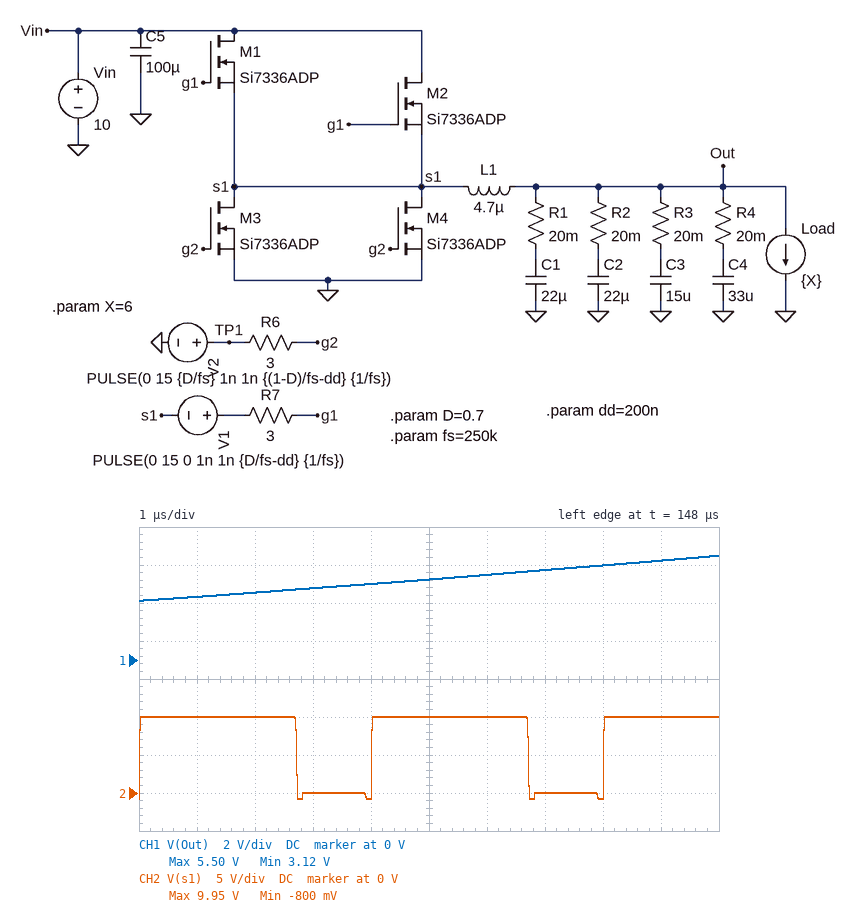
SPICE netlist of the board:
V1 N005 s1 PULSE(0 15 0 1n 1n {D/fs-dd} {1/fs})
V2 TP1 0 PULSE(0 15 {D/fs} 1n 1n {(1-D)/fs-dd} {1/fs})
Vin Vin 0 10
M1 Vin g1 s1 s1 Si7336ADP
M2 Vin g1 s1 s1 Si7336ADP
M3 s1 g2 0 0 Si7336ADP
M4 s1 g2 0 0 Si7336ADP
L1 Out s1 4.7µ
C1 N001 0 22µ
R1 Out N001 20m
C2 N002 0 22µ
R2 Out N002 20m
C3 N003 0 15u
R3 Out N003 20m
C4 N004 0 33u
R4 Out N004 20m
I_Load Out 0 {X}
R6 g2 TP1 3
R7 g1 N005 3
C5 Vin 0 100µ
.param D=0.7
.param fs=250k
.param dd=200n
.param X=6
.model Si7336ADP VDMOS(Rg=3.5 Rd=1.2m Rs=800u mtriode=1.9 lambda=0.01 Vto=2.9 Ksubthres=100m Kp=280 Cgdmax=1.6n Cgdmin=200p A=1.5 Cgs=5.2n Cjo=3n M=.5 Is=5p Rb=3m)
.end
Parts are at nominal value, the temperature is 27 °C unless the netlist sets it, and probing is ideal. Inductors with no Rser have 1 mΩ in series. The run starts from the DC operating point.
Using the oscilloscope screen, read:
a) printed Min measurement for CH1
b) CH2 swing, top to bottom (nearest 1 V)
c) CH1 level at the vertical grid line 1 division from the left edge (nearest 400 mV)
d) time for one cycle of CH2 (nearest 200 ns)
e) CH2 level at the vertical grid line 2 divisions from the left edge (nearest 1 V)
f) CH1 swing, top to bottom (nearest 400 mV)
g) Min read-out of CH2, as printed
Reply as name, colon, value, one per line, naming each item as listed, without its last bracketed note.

printed Min measurement for CH1: 3.12 V
CH2 swing, top to bottom: 11 V
CH1 level at the vertical grid line 1 division from the left edge: 3.2 V
time for one cycle of CH2: 4.0 µs
CH2 level at the vertical grid line 2 divisions from the left edge: 10 V
CH1 swing, top to bottom: 2.4 V
Min read-out of CH2, as printed: -800 mV
